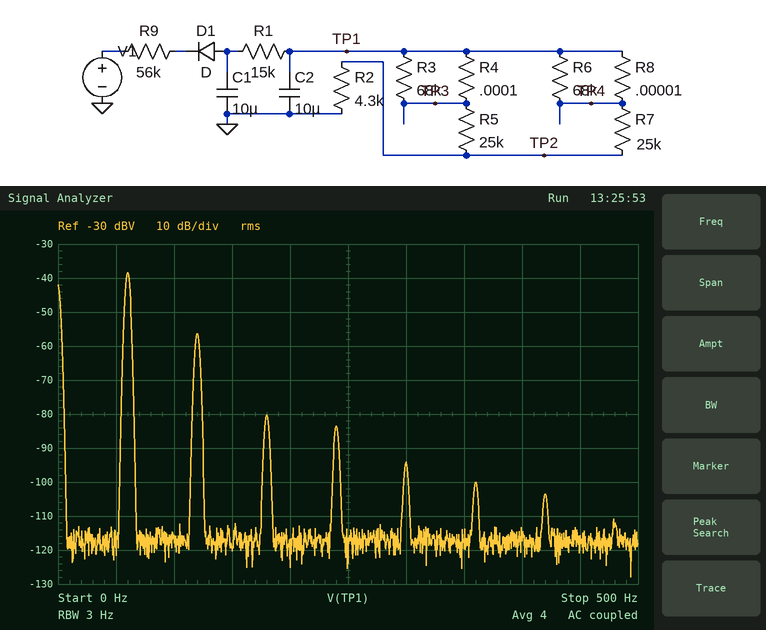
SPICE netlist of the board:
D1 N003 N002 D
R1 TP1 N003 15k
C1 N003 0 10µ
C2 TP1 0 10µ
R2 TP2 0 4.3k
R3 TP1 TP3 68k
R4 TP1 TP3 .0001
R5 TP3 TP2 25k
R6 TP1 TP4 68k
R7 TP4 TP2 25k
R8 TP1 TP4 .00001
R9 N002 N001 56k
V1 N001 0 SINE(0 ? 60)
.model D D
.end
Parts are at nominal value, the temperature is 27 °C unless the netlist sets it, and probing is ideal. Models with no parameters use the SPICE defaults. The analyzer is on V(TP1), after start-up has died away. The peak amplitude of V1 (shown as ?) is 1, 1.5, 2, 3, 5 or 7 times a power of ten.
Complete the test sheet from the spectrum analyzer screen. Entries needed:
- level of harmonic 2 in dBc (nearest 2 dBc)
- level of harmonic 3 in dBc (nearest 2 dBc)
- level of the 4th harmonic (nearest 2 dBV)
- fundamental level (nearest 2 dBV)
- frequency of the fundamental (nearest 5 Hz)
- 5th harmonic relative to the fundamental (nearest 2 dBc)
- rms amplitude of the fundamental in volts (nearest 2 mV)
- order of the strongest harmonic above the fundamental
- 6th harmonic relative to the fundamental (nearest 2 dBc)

-18 dBc
-42 dBc
-84 dBV
-38 dBV
60 Hz
-56 dBc
12 mV
2
-62 dBc
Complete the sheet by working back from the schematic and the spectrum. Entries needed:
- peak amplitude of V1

500 V
